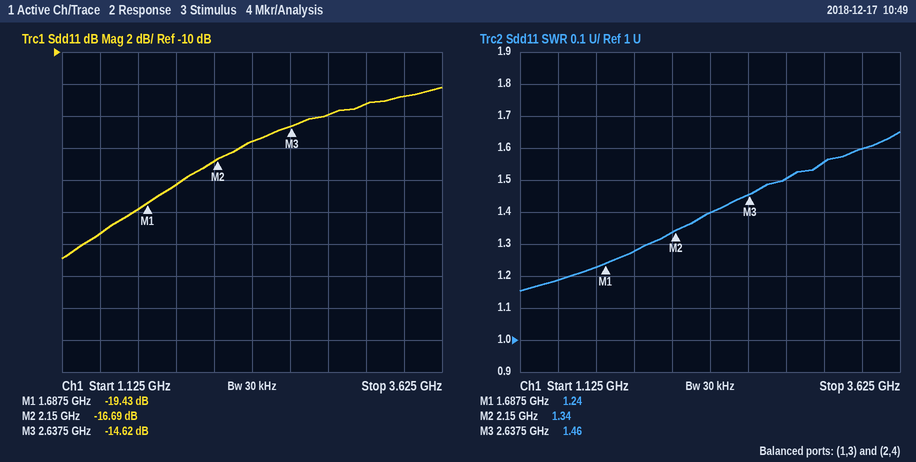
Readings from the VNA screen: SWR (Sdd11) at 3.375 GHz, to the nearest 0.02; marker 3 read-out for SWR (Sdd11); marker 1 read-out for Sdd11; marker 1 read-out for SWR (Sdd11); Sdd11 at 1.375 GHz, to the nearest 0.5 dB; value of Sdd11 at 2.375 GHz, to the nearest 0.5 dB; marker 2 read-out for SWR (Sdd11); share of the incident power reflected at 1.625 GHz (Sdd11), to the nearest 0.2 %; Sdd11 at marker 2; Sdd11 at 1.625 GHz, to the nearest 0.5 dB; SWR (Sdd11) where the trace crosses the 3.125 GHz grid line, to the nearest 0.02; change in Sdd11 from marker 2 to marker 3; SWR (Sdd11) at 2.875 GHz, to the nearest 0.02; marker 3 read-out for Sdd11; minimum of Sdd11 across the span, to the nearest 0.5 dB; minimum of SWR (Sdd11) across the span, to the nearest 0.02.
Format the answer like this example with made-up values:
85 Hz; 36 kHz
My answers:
1.60; 1.46; -19.43 dB; 1.24; -21.5 dB; -15.5 dB; 1.34; 1.0 %; -16.69 dB; -20.0 dB; 1.56; 2.07 dB; 1.50; -14.62 dB; -23.0 dB; 1.16
